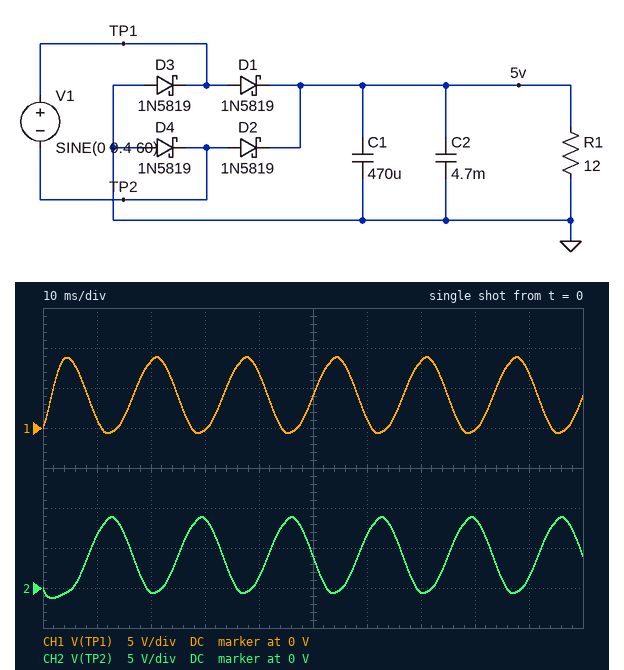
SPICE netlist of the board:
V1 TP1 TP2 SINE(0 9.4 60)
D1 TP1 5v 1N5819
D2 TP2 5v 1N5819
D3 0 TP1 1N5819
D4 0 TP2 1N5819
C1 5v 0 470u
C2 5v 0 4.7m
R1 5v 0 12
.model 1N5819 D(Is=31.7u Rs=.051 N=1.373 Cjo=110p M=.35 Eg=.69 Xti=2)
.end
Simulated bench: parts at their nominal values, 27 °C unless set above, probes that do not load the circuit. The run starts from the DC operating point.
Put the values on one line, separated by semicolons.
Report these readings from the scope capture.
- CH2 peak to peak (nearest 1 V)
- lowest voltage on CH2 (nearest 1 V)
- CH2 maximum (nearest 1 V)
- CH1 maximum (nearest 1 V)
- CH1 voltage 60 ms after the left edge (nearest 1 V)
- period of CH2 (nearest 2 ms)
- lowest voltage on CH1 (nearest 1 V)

10 V; -1 V; 9 V; 9 V; 1 V; 16 ms; -1 V
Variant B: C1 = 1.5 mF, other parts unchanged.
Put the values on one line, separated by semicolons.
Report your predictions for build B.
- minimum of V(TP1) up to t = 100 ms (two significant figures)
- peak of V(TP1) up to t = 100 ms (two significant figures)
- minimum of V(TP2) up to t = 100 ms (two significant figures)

-660 mV; 8.8 V; -1.4 V
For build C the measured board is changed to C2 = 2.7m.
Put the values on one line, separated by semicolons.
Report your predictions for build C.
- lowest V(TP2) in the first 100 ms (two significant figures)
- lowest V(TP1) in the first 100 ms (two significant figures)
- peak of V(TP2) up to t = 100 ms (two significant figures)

-960 mV; -630 mV; 8.9 V
